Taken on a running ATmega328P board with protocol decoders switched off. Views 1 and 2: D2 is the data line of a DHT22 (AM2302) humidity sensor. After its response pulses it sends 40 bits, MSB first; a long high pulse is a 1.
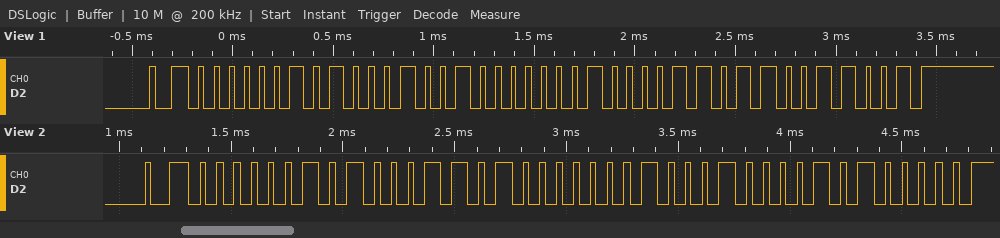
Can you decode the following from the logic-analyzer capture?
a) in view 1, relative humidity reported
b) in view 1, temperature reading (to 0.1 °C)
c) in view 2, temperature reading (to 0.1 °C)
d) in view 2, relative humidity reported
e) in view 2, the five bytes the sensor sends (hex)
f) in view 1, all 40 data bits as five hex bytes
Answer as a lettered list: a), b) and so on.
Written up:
a) 64.9 %
b) 26.9 °C
c) 27.2 °C
d) 65.3 %
e) 02 8D 01 10 A0
f) 02 89 01 0D 99
